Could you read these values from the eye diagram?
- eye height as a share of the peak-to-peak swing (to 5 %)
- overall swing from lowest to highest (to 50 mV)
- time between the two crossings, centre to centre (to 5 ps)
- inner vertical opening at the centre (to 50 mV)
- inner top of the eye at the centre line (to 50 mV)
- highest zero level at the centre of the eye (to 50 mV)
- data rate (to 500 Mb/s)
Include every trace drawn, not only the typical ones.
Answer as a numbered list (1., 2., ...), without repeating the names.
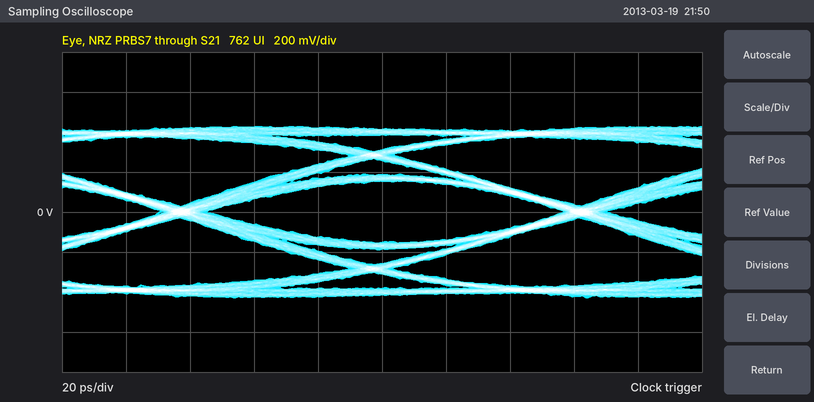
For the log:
1. 35 %
2. 850 mV
3. 125 ps
4. 300 mV
5. 150 mV
6. -150 mV
7. 8.0 Gb/s
